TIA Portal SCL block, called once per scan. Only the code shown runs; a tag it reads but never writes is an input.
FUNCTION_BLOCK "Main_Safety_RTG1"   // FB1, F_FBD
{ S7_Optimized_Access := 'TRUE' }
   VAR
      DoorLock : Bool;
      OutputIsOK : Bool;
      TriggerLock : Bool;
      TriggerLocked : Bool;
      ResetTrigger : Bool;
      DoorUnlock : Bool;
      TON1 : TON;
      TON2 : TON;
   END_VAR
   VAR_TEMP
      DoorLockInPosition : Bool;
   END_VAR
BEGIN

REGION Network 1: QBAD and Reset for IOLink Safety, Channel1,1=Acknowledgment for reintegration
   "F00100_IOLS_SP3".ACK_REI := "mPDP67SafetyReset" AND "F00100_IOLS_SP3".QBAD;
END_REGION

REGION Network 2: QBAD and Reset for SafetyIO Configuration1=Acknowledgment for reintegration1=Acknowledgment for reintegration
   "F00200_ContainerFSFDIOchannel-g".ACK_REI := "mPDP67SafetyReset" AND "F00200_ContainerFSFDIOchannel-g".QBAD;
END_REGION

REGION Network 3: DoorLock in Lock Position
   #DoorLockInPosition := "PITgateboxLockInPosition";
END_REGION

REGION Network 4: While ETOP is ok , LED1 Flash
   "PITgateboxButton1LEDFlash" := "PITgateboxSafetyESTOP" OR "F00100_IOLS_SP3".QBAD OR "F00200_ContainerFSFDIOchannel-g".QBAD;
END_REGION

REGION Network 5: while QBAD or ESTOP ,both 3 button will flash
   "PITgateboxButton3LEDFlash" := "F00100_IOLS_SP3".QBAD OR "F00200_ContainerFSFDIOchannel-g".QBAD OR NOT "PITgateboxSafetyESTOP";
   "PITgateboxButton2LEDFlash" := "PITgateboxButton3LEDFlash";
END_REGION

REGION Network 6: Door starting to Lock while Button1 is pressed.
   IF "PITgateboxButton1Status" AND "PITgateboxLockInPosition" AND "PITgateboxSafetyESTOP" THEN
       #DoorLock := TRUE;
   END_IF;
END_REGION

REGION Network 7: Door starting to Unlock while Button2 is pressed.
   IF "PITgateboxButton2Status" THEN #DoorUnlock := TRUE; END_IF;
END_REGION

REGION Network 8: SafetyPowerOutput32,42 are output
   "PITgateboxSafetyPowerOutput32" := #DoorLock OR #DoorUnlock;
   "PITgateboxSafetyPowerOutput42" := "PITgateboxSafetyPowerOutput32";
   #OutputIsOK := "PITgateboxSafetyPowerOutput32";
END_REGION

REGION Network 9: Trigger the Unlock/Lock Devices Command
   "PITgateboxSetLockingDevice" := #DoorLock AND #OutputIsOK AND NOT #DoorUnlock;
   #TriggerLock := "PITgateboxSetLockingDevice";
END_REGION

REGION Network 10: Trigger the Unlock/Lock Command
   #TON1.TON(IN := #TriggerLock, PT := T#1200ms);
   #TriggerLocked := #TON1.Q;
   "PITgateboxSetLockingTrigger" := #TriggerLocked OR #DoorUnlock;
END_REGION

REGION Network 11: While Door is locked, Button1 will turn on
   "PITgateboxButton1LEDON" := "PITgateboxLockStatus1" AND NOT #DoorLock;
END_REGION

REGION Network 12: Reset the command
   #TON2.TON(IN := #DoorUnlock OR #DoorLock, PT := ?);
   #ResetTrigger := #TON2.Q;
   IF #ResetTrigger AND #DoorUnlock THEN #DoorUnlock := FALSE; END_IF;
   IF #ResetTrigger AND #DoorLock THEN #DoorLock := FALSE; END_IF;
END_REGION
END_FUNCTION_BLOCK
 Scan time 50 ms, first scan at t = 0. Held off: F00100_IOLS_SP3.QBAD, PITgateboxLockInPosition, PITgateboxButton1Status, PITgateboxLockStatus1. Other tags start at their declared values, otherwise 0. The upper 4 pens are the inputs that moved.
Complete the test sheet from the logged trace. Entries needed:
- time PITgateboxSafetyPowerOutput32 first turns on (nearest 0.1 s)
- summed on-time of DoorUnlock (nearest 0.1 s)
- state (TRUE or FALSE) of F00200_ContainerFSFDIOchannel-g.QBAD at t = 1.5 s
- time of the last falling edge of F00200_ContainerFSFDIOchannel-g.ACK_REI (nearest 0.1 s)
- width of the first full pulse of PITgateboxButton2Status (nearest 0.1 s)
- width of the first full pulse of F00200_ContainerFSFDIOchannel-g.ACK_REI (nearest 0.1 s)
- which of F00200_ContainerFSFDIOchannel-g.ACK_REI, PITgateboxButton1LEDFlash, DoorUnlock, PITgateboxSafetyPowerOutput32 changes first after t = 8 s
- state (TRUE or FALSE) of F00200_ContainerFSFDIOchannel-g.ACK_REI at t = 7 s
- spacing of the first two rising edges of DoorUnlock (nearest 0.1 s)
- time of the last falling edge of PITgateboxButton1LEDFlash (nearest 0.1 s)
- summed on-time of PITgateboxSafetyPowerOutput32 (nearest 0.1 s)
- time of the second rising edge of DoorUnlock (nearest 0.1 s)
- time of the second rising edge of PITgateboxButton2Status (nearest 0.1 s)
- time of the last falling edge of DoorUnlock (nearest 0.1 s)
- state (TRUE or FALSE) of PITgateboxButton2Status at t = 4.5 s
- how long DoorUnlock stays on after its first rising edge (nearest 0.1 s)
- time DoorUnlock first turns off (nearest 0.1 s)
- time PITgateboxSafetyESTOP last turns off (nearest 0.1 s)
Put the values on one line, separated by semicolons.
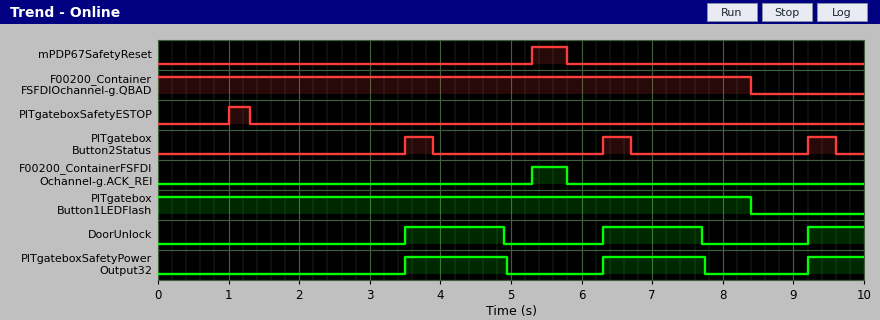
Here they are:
3.5 s; 3.6 s; TRUE; 5.8 s; 0.4 s; 0.5 s; PITgateboxButton1LEDFlash; FALSE; 2.8 s; 8.4 s; 3.7 s; 6.3 s; 6.3 s; 7.7 s; FALSE; 1.4 s; 4.9 s; 1.3 s
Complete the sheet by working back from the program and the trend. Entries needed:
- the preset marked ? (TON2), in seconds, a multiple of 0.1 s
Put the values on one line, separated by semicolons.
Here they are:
1.4 s
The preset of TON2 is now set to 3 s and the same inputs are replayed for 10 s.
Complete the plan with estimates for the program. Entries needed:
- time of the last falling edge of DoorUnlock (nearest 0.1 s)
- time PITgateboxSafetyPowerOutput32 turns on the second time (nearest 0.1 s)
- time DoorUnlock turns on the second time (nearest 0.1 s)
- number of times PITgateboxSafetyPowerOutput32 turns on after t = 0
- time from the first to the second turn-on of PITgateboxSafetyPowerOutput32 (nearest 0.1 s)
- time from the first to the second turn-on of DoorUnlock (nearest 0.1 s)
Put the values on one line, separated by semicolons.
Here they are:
6.5 s; 9.2 s; 9.2 s; 2; 5.7 s; 5.7 s
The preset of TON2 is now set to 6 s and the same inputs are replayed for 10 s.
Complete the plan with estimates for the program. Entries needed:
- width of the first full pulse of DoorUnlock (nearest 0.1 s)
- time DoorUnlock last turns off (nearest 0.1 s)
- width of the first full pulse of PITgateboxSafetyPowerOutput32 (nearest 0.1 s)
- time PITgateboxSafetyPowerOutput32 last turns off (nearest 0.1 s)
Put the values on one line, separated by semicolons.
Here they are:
6.0 s; 9.5 s; 6.1 s; 9.6 s
